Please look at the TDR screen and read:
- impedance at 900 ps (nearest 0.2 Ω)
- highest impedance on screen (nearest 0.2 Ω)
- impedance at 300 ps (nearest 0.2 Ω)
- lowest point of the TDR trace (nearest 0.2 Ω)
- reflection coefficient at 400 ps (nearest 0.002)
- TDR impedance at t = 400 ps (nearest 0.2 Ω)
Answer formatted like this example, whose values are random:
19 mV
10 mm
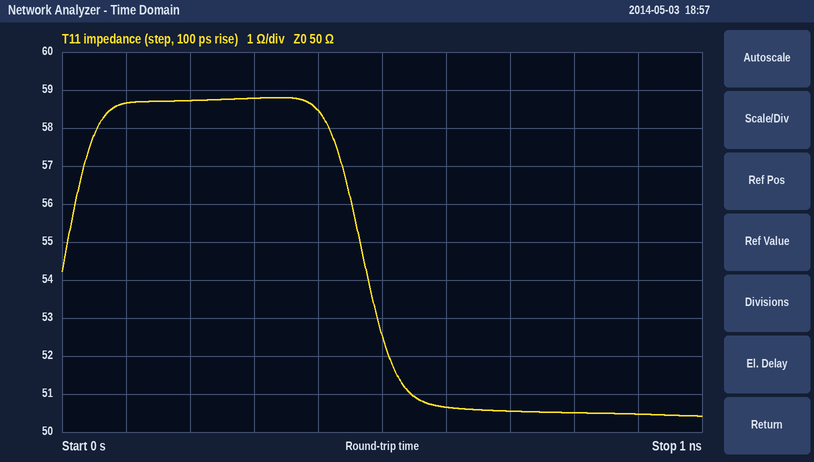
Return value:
50.4 Ω
58.8 Ω
58.8 Ω
50.4 Ω
+0.078
58.4 Ω
